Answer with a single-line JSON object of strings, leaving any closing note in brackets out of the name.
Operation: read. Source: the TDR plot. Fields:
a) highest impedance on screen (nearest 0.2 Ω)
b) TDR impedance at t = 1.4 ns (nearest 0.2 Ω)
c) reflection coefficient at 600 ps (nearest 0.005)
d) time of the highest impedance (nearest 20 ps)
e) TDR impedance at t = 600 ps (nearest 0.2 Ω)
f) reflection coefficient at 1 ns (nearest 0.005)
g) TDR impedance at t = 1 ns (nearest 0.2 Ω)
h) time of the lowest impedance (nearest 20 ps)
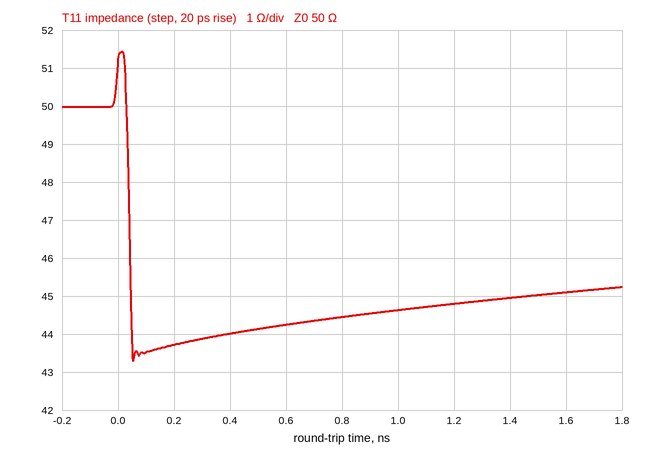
{"highest impedance on screen": "51.4 Ω", "TDR impedance at t = 1.4 ns": "45.0 Ω", "reflection coefficient at 600 ps": "-0.060", "time of the highest impedance": "20 ps", "TDR impedance at t = 600 ps": "44.2 Ω", "reflection coefficient at 1 ns": "-0.055", "TDR impedance at t = 1 ns": "44.6 Ω", "time of the lowest impedance": "60 ps"}
